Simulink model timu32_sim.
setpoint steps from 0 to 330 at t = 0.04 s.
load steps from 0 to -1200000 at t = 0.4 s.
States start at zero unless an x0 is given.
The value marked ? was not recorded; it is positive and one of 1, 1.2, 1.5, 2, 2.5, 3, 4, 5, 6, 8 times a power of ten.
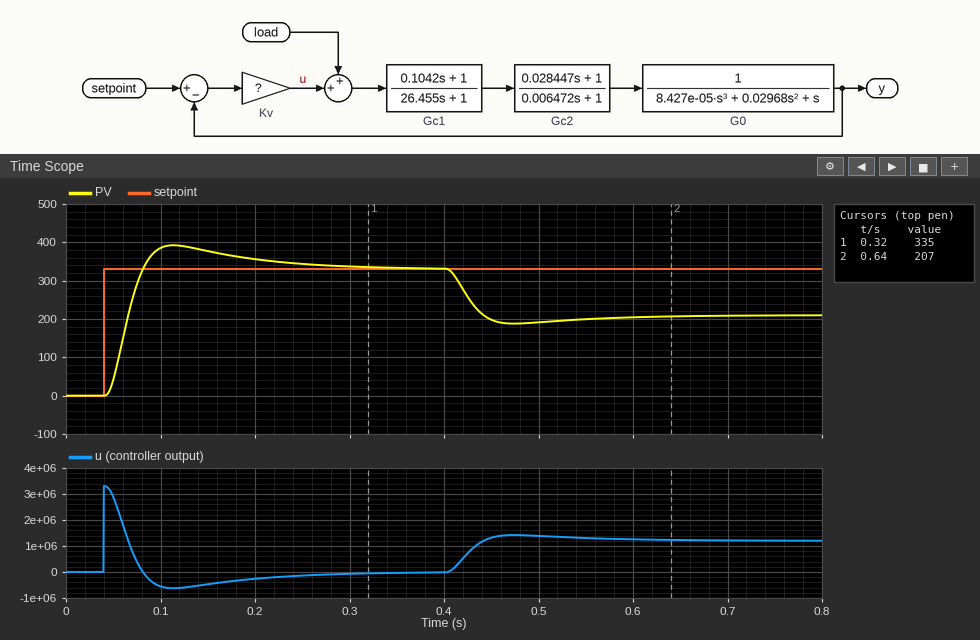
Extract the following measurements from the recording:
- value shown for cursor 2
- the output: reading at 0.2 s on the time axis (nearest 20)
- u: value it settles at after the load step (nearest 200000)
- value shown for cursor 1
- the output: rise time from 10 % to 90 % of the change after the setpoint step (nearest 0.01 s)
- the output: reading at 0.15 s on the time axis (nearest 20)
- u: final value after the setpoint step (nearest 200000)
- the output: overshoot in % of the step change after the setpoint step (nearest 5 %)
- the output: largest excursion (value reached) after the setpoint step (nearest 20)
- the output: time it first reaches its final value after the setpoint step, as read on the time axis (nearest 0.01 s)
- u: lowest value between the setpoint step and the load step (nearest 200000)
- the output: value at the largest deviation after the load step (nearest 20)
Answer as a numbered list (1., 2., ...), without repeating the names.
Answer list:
1. 207
2. 360
3. 1200000
4. 335
5. 0.03 s
6. 380
7. 0
8. 20 %
9. 400
10. 0.08 s
11. -600000
12. 180
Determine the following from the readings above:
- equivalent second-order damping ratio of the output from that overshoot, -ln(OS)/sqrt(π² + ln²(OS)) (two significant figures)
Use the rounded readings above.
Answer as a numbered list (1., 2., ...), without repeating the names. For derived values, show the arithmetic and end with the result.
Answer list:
1. ln(0.2) = -1.609; 1.609 / sqrt(9.870 + 2.590) = 0.46
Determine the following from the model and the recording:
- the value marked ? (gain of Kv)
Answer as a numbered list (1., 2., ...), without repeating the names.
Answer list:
1. 10000
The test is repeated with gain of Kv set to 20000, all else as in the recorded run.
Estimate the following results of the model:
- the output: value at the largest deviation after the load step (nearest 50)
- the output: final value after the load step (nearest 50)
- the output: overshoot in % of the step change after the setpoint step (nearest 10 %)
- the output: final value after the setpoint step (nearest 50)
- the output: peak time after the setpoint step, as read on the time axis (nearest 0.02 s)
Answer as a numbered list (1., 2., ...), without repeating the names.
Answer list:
1. 250
2. 250
3. 30 %
4. 350
5. 0.08 s
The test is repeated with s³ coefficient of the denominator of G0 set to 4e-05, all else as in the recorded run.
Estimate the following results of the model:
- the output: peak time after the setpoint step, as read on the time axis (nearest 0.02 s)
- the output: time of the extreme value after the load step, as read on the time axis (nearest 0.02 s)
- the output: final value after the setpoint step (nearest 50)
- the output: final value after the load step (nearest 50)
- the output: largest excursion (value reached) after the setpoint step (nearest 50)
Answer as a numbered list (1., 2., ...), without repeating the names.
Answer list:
1. 0.12 s
2. 0.48 s
3. 350
4. 200
5. 400
